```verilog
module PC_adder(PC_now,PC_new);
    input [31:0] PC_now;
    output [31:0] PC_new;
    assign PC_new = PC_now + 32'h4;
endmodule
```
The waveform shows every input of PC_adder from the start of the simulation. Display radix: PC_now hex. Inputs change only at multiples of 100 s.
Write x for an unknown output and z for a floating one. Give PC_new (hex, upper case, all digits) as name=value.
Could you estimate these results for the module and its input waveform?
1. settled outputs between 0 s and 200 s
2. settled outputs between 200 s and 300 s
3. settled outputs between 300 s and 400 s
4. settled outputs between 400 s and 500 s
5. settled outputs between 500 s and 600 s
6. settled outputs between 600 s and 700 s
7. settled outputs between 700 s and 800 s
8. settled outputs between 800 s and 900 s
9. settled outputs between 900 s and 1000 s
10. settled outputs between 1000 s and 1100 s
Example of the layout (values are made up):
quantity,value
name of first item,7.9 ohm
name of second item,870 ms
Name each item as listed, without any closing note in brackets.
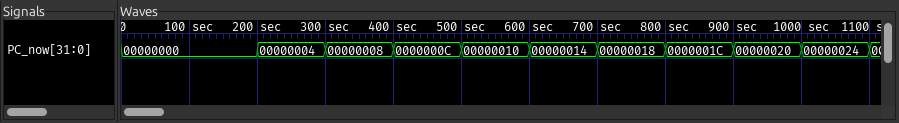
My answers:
quantity,value
settled outputs between 0 s and 200 s,PC_new=00000004
settled outputs between 200 s and 300 s,PC_new=00000008
settled outputs between 300 s and 400 s,PC_new=0000000C
settled outputs between 400 s and 500 s,PC_new=00000010
settled outputs between 500 s and 600 s,PC_new=00000014
settled outputs between 600 s and 700 s,PC_new=00000018
settled outputs between 700 s and 800 s,PC_new=0000001C
settled outputs between 800 s and 900 s,PC_new=00000020
settled outputs between 900 s and 1000 s,PC_new=00000024
settled outputs between 1000 s and 1100 s,PC_new=00000028
